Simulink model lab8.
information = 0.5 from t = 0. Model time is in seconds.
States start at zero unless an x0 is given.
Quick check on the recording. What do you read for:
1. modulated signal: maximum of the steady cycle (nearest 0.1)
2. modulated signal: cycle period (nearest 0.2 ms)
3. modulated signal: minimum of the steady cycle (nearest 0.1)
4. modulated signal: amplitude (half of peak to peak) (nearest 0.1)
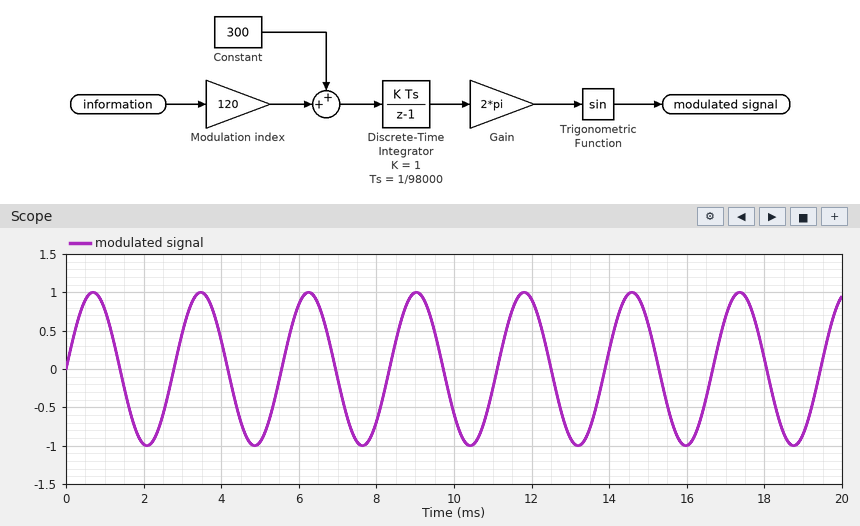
1.0
2.8 ms
-1.0
1.0
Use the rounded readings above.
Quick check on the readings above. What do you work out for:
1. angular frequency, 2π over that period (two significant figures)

2.2 rad/ms
